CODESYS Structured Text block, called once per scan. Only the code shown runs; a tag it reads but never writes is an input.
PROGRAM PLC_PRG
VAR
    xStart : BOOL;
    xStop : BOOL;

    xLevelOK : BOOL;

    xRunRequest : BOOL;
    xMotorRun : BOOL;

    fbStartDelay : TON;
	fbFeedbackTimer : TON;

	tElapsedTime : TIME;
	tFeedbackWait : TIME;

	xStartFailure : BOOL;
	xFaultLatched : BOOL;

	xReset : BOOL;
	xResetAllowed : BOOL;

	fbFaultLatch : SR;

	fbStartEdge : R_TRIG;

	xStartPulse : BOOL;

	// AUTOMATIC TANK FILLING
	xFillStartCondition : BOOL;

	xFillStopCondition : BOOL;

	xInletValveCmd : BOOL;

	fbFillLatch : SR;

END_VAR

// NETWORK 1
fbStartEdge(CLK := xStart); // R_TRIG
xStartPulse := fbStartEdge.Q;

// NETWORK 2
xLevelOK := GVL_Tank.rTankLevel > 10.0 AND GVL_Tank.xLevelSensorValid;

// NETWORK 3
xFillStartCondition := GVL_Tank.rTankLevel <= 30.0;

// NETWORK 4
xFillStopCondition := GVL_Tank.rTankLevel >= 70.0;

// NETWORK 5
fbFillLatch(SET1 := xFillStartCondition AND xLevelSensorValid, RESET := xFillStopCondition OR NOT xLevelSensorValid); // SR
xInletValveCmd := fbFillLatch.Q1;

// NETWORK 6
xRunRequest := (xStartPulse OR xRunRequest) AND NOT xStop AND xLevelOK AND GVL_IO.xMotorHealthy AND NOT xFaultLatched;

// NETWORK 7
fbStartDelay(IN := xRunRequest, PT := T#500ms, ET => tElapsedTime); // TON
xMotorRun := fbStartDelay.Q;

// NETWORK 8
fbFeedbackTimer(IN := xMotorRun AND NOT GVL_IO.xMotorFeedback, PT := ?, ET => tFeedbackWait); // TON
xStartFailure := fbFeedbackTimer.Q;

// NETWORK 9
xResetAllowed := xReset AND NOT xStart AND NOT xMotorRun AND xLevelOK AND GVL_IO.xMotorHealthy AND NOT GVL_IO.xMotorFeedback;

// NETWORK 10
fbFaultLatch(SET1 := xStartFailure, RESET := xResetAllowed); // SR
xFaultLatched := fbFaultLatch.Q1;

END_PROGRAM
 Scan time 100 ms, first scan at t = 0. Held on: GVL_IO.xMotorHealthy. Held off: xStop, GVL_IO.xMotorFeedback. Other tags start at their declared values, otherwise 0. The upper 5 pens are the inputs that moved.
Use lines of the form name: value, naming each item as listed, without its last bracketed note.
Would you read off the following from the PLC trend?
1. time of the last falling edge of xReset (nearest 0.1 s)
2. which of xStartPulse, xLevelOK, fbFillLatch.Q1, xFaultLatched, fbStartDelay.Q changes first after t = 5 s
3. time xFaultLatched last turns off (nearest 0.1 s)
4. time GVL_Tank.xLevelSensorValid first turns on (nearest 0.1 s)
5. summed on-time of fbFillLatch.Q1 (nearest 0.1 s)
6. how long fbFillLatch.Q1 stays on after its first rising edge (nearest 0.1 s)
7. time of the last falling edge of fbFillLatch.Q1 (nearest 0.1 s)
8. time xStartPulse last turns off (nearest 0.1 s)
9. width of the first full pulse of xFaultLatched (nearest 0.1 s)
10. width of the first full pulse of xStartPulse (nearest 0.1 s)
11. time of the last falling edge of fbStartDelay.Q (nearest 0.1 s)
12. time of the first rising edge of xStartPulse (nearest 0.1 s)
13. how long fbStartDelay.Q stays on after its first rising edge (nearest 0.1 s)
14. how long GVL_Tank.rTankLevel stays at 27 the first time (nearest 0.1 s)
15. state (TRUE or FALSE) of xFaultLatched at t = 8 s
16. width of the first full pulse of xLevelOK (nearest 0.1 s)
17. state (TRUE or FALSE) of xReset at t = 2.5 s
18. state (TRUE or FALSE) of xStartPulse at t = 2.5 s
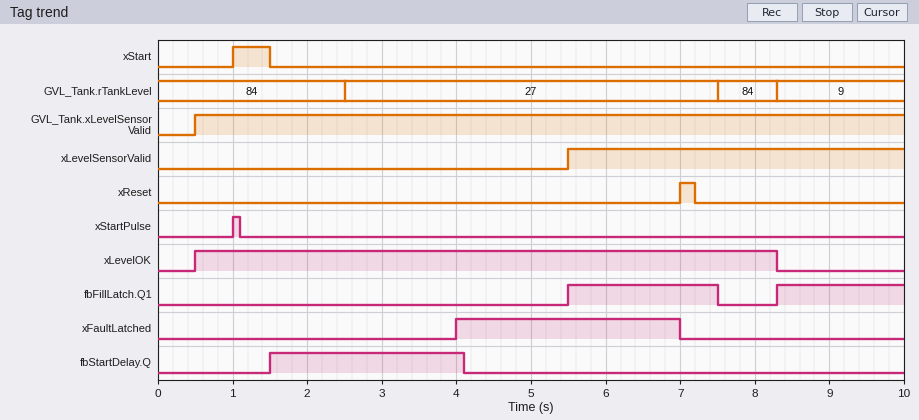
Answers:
time of the last falling edge of xReset: 7.2 s
which of xStartPulse, xLevelOK, fbFillLatch.Q1, xFaultLatched, fbStartDelay.Q changes first after t = 5 s: fbFillLatch.Q1
time xFaultLatched last turns off: 7.0 s
time GVL_Tank.xLevelSensorValid first turns on: 0.5 s
summed on-time of fbFillLatch.Q1: 3.7 s
how long fbFillLatch.Q1 stays on after its first rising edge: 2.0 s
time of the last falling edge of fbFillLatch.Q1: 7.5 s
time xStartPulse last turns off: 1.1 s
width of the first full pulse of xFaultLatched: 3.0 s
width of the first full pulse of xStartPulse: 0.1 s
time of the last falling edge of fbStartDelay.Q: 4.1 s
time of the first rising edge of xStartPulse: 1.0 s
how long fbStartDelay.Q stays on after its first rising edge: 2.6 s
how long GVL_Tank.rTankLevel stays at 27 the first time: 5.0 s
state (TRUE or FALSE) of xFaultLatched at t = 8 s: FALSE
width of the first full pulse of xLevelOK: 7.8 s
state (TRUE or FALSE) of xReset at t = 2.5 s: FALSE
state (TRUE or FALSE) of xStartPulse at t = 2.5 s: FALSE
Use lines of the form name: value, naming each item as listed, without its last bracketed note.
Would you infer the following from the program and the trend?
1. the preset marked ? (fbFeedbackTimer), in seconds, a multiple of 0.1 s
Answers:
the preset marked ? (fbFeedbackTimer), in seconds, a multiple of 0.1 s: 2.5 s
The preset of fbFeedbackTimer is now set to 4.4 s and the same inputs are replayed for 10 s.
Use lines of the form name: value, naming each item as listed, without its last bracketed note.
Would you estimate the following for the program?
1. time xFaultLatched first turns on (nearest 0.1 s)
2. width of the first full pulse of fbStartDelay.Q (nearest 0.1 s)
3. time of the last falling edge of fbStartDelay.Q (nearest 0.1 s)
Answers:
time xFaultLatched first turns on: 5.9 s
width of the first full pulse of fbStartDelay.Q: 4.5 s
time of the last falling edge of fbStartDelay.Q: 6.0 s
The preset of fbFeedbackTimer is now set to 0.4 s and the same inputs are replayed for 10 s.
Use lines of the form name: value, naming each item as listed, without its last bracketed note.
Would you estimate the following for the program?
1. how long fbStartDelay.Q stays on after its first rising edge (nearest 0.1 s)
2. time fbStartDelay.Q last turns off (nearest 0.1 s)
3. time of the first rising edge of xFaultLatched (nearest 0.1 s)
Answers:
how long fbStartDelay.Q stays on after its first rising edge: 0.5 s
time fbStartDelay.Q last turns off: 2.0 s
time of the first rising edge of xFaultLatched: 1.9 s
